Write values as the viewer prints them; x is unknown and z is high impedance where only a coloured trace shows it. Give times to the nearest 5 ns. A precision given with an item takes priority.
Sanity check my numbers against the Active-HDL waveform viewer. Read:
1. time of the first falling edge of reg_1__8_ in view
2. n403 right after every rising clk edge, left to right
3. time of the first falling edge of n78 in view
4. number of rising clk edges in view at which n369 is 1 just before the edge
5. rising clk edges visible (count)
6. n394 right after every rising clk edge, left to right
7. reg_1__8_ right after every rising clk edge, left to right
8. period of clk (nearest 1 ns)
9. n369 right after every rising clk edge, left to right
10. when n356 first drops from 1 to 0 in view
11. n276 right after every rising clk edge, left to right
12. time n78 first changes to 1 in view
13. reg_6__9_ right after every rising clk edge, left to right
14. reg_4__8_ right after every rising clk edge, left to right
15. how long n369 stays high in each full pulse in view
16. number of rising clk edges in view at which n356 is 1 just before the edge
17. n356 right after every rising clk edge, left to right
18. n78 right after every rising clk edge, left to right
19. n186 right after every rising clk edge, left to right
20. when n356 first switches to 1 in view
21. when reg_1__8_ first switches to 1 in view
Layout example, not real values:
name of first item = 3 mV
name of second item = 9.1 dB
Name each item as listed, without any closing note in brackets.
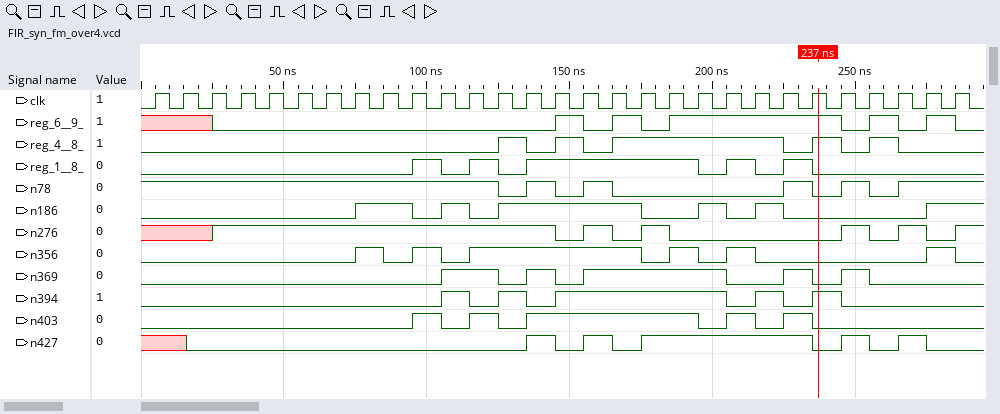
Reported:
time of the first falling edge of reg_1__8_ in view = 105 ns
n403 right after every rising clk edge, left to right = 0 0 0 0 0 0 0 0 0 1 0 1 0 1 1 1 1 1 1 0 1 0 1 0 0 0 0 0 0
time of the first falling edge of n78 in view = 125 ns
number of rising clk edges in view at which n369 is 1 just before the edge = 10
rising clk edges visible = 29
n394 right after every rising clk edge, left to right = 0 0 0 0 0 0 0 0 0 0 1 0 1 0 1 1 1 1 1 1 0 1 0 1 0 0 0 0 0
reg_1__8_ right after every rising clk edge, left to right = 0 0 0 0 0 0 0 0 0 1 0 1 0 1 1 1 1 1 1 0 1 0 1 0 0 0 0 0 0
period of clk = 10 ns
n369 right after every rising clk edge, left to right = 0 0 0 0 0 0 0 0 0 0 1 1 0 1 0 1 1 1 1 1 0 0 1 0 1 0 0 0 0
when n356 first drops from 1 to 0 in view = 85 ns
n276 right after every rising clk edge, left to right = x x 1 1 1 1 1 1 1 1 1 1 1 1 0 1 0 1 0 0 0 0 0 0 1 0 1 0 1
time n78 first changes to 1 in view = 135 ns
reg_6__9_ right after every rising clk edge, left to right = x x 0 0 0 0 0 0 0 0 0 0 0 0 1 0 1 0 1 1 1 1 1 1 0 1 0 1 0
reg_4__8_ right after every rising clk edge, left to right = 0 0 0 0 0 0 0 0 0 0 0 0 1 0 1 0 1 1 1 1 1 1 0 1 0 1 0 0 0
how long n369 stays high in each full pulse in view = 20 ns, 10 ns, 50 ns, 10 ns, 10 ns
number of rising clk edges in view at which n356 is 1 just before the edge = 11
n356 right after every rising clk edge, left to right = 0 0 0 0 0 0 0 1 0 1 0 1 1 1 1 1 1 0 1 0 1 0 0 0 0 0 0 1 0
n78 right after every rising clk edge, left to right = 1 1 1 1 1 1 1 1 1 1 1 1 0 1 0 1 0 0 0 0 0 0 1 0 1 0 1 1 1
n186 right after every rising clk edge, left to right = 0 0 0 0 0 0 0 1 1 0 1 0 1 1 1 1 1 0 0 1 0 1 0 0 0 0 0 1 1
when n356 first switches to 1 in view = 75 ns
when reg_1__8_ first switches to 1 in view = 95 ns
